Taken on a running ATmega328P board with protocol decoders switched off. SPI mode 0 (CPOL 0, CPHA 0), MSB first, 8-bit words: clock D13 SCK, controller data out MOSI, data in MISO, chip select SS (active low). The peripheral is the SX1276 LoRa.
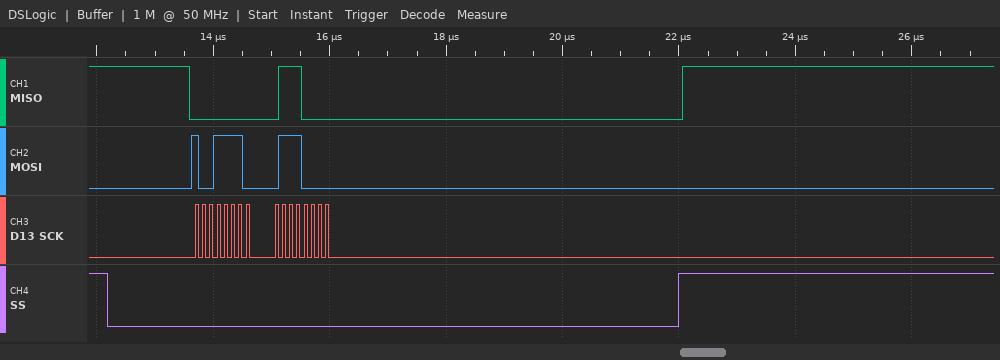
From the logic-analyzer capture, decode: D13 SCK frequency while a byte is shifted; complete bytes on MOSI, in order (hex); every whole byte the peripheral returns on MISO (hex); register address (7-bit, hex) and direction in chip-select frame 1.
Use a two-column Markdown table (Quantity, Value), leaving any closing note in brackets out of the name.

| Quantity | Value |
|---|---|
| D13 SCK frequency while a byte is shifted | 8 MHz |
| complete bytes on MOSI, in order | 9E 70 |
| every whole byte the peripheral returns on MISO | 00 70 |
| register address (7-bit, hex) and direction in chip-select frame 1 | 0x1E write |
